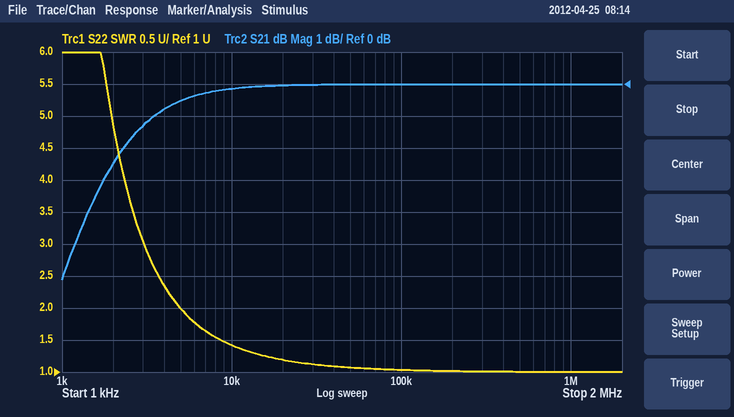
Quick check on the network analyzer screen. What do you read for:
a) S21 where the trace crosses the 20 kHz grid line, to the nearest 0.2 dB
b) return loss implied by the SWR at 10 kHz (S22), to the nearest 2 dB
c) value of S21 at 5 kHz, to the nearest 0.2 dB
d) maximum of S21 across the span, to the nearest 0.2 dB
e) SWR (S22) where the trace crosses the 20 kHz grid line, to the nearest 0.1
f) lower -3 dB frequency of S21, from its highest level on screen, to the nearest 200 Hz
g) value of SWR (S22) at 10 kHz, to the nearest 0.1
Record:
0.0 dB
16 dB
-0.6 dB
0.0 dB
1.2
1.8 kHz
1.4
